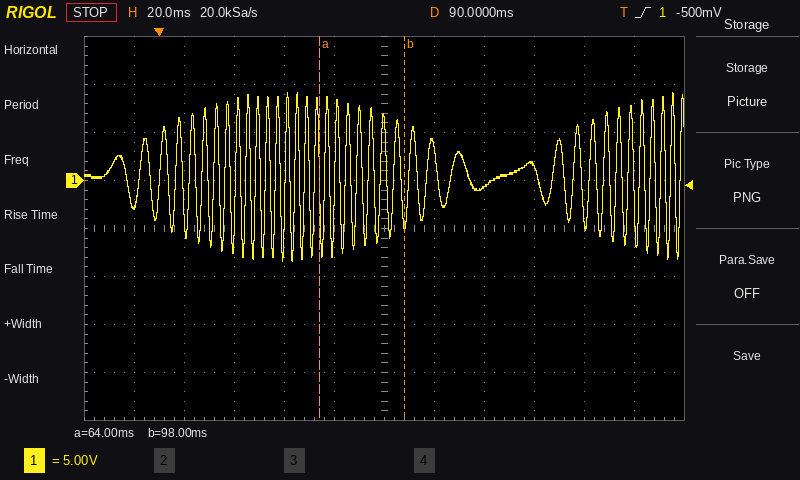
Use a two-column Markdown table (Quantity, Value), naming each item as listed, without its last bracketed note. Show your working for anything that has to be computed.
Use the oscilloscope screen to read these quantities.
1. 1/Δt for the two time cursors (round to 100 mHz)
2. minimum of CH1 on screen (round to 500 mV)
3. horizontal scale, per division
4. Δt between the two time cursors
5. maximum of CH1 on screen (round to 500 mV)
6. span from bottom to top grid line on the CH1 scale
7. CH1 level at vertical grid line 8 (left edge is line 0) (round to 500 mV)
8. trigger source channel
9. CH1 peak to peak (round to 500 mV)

| Quantity | Value |
|---|---|
| 1/Δt for the two time cursors | 1 / 34 ms ≈ 29.4 Hz |
| minimum of CH1 on screen | -8.5 V |
| horizontal scale, per division | 20 ms |
| Δt between the two time cursors | 98 ms − (64 ms) = 34 ms |
| maximum of CH1 on screen | 9.0 V |
| span from bottom to top grid line on the CH1 scale | 40 V |
| CH1 level at vertical grid line 8 (left edge is line 0) | -500 mV |
| trigger source channel | CH1 |
| CH1 peak to peak | 9.0 V − (-8.5 V) = 17.5 V |
